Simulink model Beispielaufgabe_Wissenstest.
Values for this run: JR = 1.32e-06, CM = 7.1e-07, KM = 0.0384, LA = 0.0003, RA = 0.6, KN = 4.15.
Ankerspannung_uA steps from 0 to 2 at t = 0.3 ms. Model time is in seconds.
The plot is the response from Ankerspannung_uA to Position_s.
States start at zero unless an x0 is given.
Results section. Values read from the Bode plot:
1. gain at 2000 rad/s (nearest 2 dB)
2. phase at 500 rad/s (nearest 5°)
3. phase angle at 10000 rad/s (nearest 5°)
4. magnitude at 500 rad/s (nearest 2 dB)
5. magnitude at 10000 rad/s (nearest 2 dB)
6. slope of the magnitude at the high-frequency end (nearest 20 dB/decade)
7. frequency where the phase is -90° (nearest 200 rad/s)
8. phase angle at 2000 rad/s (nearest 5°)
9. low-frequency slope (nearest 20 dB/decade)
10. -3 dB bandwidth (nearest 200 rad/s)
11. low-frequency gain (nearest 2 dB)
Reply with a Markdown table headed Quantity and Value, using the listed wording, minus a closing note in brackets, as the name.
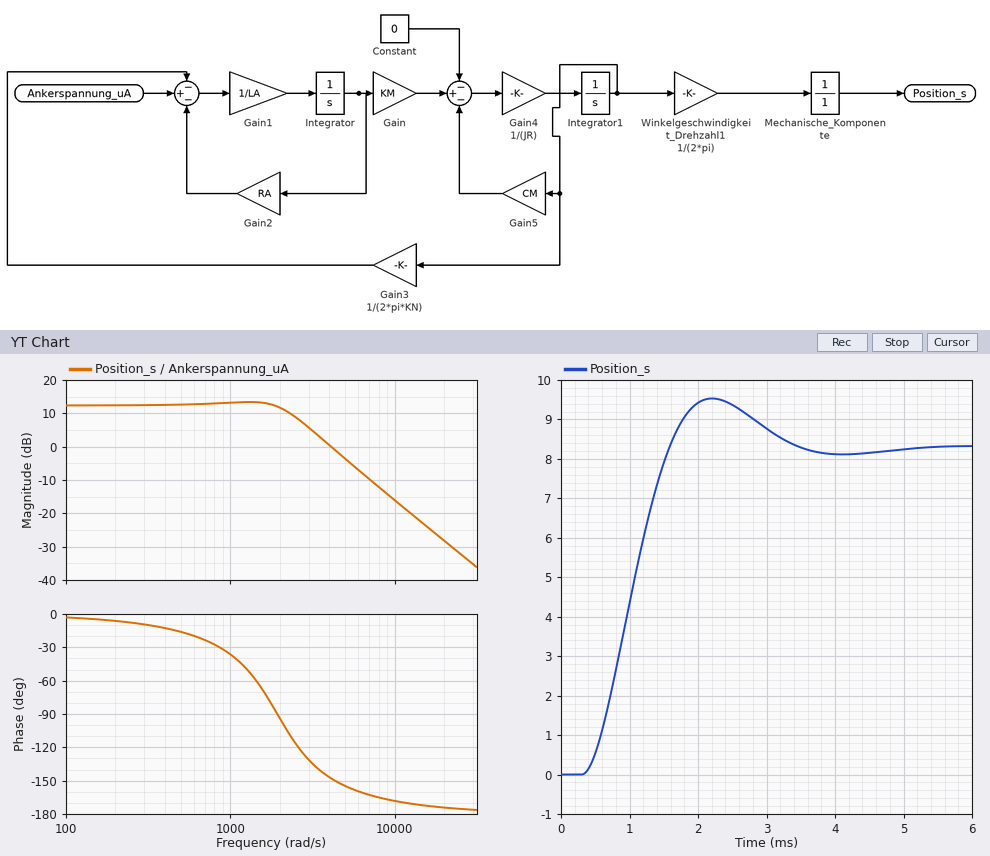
| Quantity | Value |
|---|---|
| gain at 2000 rad/s | 12 dB |
| phase at 500 rad/s | -15° |
| phase angle at 10000 rad/s | -170° |
| magnitude at 500 rad/s | 12 dB |
| magnitude at 10000 rad/s | -16 dB |
| slope of the magnitude at the high-frequency end | -40 dB/decade |
| frequency where the phase is -90° | 2000 rad/s |
| phase angle at 2000 rad/s | -95° |
| low-frequency slope | 0 dB/decade |
| -3 dB bandwidth | 2400 rad/s |
| low-frequency gain | 12 dB |
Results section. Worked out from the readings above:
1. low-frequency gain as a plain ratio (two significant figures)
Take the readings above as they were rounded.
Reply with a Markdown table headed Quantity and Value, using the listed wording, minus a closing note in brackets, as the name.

| Quantity | Value |
|---|---|
| low-frequency gain as a plain ratio | 4.0 |
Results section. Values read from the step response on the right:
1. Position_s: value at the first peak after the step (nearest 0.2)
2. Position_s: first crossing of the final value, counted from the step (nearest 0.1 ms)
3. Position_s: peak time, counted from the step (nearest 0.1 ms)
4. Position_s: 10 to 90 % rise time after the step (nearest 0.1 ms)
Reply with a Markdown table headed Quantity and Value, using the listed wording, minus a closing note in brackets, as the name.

| Quantity | Value |
|---|---|
| Position_s: value at the first peak after the step | 9.6 |
| Position_s: first crossing of the final value, counted from the step | 1.3 ms |
| Position_s: peak time, counted from the step | 1.9 ms |
| Position_s: 10 to 90 % rise time after the step | 0.9 ms |
